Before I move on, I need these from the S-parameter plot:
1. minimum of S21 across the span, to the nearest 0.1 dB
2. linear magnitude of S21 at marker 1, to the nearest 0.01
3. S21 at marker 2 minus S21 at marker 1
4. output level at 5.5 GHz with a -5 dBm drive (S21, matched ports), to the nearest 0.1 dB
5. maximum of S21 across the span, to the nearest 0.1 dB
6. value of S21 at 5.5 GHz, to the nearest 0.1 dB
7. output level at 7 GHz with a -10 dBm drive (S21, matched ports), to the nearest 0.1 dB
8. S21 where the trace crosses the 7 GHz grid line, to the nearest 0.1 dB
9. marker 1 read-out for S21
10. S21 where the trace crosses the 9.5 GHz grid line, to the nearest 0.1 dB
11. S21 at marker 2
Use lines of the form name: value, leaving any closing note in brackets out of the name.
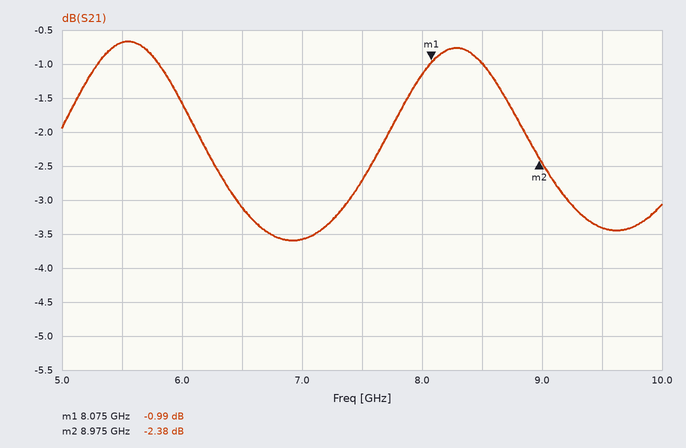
minimum of S21 across the span, to the nearest 0.1 dB: -3.6 dB
linear magnitude of S21 at marker 1, to the nearest 0.01: 0.89
S21 at marker 2 minus S21 at marker 1: -1.39 dB
output level at 5.5 GHz with a -5 dBm drive (S21, matched ports), to the nearest 0.1 dB: -5.7 dBm
maximum of S21 across the span, to the nearest 0.1 dB: -0.7 dB
value of S21 at 5.5 GHz, to the nearest 0.1 dB: -0.7 dB
output level at 7 GHz with a -10 dBm drive (S21, matched ports), to the nearest 0.1 dB: -13.6 dBm
S21 where the trace crosses the 7 GHz grid line, to the nearest 0.1 dB: -3.6 dB
marker 1 read-out for S21: -0.99 dB
S21 where the trace crosses the 9.5 GHz grid line, to the nearest 0.1 dB: -3.4 dB
S21 at marker 2: -2.38 dB
